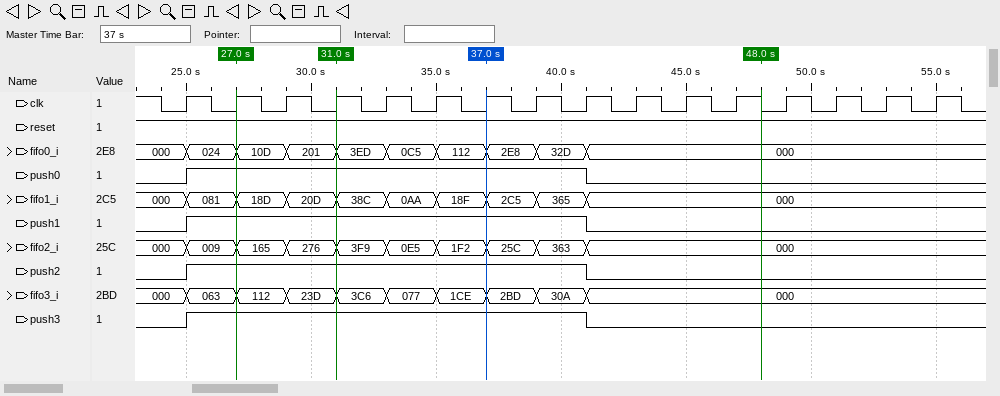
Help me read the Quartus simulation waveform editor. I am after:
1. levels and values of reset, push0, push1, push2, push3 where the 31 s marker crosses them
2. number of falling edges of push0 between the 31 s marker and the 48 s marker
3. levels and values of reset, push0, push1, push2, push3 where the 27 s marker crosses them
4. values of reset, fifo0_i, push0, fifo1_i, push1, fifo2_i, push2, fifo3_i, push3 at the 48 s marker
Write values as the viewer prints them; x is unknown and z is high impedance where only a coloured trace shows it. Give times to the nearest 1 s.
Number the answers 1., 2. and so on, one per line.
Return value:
1. reset=1, push0=1, push1=1, push2=1, push3=1
2. 1
3. reset=1, push0=1, push1=1, push2=1, push3=1
4. reset=1, fifo0_i=000, push0=0, fifo1_i=000, push1=0, fifo2_i=000, push2=0, fifo3_i=000, push3=0
